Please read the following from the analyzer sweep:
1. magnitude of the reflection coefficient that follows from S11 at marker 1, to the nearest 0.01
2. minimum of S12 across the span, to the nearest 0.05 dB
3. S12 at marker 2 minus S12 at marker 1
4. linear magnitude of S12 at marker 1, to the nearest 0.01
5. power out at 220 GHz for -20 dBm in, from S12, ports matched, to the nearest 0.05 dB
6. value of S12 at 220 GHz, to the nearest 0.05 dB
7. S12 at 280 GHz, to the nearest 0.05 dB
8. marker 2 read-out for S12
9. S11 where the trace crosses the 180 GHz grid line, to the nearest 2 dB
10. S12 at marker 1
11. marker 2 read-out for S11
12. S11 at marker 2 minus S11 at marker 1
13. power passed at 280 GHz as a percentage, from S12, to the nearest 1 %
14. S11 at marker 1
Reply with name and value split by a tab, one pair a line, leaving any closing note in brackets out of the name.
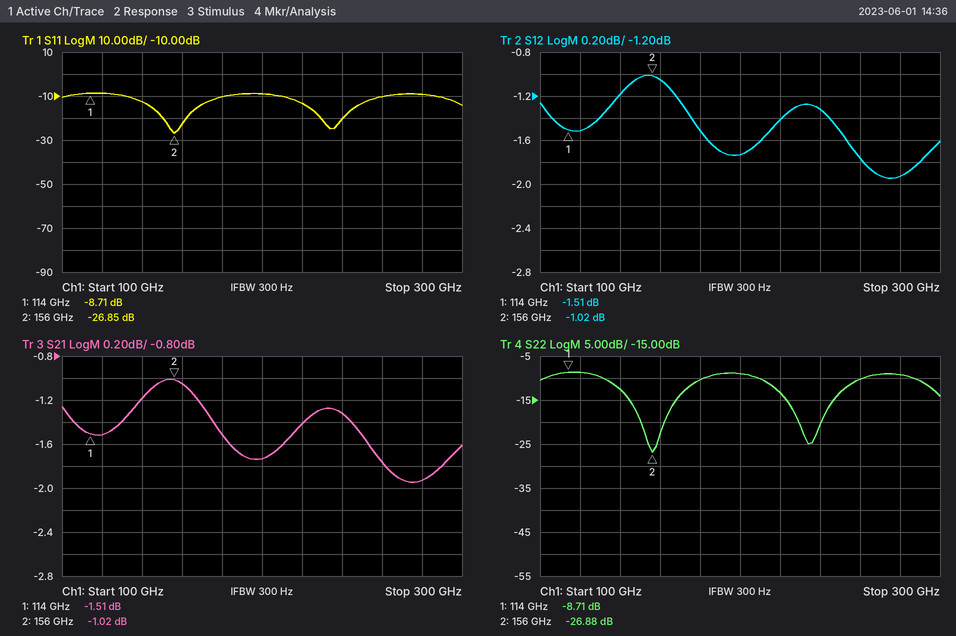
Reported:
magnitude of the reflection coefficient that follows from S11 at marker 1, to the nearest 0.01	0.37
minimum of S12 across the span, to the nearest 0.05 dB	-1.95 dB
S12 at marker 2 minus S12 at marker 1	0.49 dB
linear magnitude of S12 at marker 1, to the nearest 0.01	0.84
power out at 220 GHz for -20 dBm in, from S12, ports matched, to the nearest 0.05 dB	-21.40 dBm
value of S12 at 220 GHz, to the nearest 0.05 dB	-1.40 dB
S12 at 280 GHz, to the nearest 0.05 dB	-1.95 dB
marker 2 read-out for S12	-1.02 dB
S11 where the trace crosses the 180 GHz grid line, to the nearest 2 dB	-10 dB
S12 at marker 1	-1.51 dB
marker 2 read-out for S11	-26.85 dB
S11 at marker 2 minus S11 at marker 1	-18.14 dB
power passed at 280 GHz as a percentage, from S12, to the nearest 1 %	64 %
S11 at marker 1	-8.71 dB
